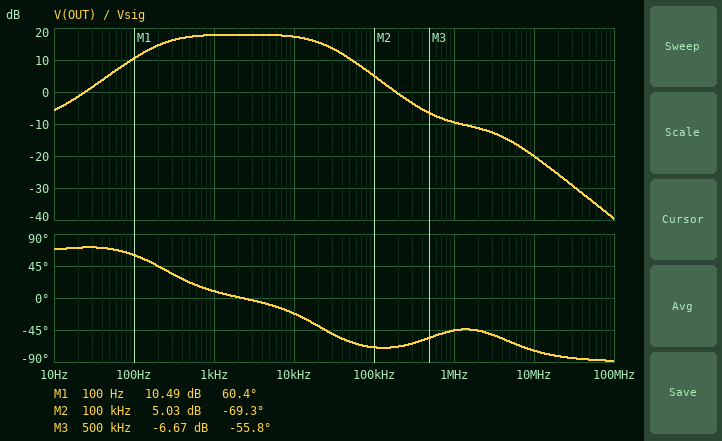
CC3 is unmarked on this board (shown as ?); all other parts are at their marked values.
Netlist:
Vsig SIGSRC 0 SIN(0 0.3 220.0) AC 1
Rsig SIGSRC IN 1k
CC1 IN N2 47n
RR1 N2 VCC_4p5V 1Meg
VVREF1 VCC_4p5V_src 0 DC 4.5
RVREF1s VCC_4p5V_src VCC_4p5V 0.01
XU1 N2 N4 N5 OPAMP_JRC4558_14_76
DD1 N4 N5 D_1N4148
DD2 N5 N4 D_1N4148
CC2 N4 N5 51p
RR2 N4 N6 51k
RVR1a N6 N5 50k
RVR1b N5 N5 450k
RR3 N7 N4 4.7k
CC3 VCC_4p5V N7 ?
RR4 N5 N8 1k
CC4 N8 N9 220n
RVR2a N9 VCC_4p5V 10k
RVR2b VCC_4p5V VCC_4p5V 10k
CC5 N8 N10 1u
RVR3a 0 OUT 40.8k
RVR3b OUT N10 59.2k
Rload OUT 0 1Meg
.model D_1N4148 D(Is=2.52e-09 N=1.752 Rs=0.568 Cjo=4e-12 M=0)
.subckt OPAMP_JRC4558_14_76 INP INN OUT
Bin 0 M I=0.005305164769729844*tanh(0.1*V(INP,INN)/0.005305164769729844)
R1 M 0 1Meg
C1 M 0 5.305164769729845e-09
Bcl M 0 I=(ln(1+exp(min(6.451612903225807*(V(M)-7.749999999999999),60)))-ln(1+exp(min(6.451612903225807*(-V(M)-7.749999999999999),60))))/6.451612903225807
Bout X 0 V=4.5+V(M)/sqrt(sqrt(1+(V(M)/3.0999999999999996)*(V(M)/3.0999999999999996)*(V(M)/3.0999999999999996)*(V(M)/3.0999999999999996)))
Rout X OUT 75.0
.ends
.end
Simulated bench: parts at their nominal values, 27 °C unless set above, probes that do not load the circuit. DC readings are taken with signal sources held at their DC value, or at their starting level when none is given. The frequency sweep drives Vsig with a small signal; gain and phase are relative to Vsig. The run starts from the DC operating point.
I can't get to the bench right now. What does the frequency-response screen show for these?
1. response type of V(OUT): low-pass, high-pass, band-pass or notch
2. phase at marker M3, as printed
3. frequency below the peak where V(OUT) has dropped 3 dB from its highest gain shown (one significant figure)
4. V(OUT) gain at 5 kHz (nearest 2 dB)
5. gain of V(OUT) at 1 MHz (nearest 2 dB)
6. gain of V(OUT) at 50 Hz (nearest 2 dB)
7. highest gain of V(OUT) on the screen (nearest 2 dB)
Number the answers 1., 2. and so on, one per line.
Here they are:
1. band-pass
2. -55.8 deg
3. 200 Hz
4. 18 dB
5. -10 dB
6. 6 dB
7. 18 dB
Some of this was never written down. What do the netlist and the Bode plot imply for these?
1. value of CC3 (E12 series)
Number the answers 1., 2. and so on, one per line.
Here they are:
1. 150 nF
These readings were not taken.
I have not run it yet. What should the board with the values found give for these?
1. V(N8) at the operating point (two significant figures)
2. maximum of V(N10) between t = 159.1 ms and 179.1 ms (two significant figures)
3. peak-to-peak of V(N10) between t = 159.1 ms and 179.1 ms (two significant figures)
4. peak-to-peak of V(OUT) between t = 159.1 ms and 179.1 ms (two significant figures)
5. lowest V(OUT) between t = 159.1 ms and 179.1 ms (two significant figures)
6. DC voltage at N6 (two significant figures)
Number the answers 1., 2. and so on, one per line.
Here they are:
1. 4.5 V
2. 660 mV
3. 1.3 V
4. 530 mV
5. -260 mV
6. 4.5 V
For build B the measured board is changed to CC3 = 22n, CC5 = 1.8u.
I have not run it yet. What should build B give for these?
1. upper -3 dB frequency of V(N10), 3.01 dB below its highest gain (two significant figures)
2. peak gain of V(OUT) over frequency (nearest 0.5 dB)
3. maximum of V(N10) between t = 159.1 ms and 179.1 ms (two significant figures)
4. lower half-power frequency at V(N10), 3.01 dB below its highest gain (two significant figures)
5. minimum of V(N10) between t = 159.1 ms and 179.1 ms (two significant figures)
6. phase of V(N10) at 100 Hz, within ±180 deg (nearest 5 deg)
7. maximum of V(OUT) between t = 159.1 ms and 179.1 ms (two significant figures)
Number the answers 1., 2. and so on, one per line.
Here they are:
1. 25 kHz
2. 17.5 dB
3. 520 mV
4. 1.4 kHz
5. -520 mV
6. 50 deg
7. 210 mV
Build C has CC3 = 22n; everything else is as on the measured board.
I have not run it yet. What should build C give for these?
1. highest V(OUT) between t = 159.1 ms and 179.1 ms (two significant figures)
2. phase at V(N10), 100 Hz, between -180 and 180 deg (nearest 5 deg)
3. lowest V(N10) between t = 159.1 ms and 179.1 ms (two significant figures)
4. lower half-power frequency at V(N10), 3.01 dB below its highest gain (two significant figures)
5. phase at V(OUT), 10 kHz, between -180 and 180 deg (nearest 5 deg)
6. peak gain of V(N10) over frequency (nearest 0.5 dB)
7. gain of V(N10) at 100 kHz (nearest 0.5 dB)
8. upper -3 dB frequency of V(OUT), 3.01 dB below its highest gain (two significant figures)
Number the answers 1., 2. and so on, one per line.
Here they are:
1. 210 mV
2. 50 deg
3. -520 mV
4. 1.4 kHz
5. -15 deg
6. 25.5 dB
7. 13.0 dB
8. 25 kHz
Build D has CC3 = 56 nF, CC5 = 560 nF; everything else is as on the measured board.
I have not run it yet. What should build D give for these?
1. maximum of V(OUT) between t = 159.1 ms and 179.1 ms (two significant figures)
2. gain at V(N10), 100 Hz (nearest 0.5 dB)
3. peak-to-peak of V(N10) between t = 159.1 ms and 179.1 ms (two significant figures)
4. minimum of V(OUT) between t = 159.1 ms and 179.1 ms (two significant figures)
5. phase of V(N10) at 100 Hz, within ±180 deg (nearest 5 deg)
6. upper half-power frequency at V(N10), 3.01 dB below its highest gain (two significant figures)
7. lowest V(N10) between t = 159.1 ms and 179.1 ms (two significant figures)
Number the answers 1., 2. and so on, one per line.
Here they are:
1. 240 mV
2. 11.0 dB
3. 1.2 V
4. -240 mV
5. 65 deg
6. 24 kHz
7. -600 mV
